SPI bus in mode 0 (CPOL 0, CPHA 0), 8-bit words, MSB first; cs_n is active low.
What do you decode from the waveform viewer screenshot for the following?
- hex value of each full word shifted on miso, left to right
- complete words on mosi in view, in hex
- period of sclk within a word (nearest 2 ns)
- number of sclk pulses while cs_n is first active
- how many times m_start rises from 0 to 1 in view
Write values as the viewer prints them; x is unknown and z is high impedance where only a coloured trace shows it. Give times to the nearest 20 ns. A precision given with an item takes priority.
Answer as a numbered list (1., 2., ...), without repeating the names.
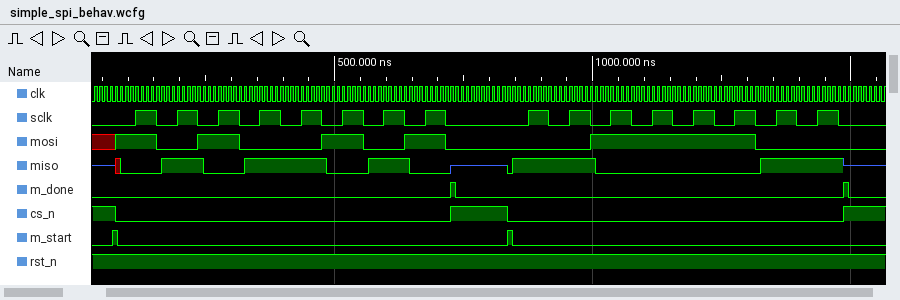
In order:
1. 5A, C3
2. A5, 3C
3. 80 ns
4. 8
5. 2
